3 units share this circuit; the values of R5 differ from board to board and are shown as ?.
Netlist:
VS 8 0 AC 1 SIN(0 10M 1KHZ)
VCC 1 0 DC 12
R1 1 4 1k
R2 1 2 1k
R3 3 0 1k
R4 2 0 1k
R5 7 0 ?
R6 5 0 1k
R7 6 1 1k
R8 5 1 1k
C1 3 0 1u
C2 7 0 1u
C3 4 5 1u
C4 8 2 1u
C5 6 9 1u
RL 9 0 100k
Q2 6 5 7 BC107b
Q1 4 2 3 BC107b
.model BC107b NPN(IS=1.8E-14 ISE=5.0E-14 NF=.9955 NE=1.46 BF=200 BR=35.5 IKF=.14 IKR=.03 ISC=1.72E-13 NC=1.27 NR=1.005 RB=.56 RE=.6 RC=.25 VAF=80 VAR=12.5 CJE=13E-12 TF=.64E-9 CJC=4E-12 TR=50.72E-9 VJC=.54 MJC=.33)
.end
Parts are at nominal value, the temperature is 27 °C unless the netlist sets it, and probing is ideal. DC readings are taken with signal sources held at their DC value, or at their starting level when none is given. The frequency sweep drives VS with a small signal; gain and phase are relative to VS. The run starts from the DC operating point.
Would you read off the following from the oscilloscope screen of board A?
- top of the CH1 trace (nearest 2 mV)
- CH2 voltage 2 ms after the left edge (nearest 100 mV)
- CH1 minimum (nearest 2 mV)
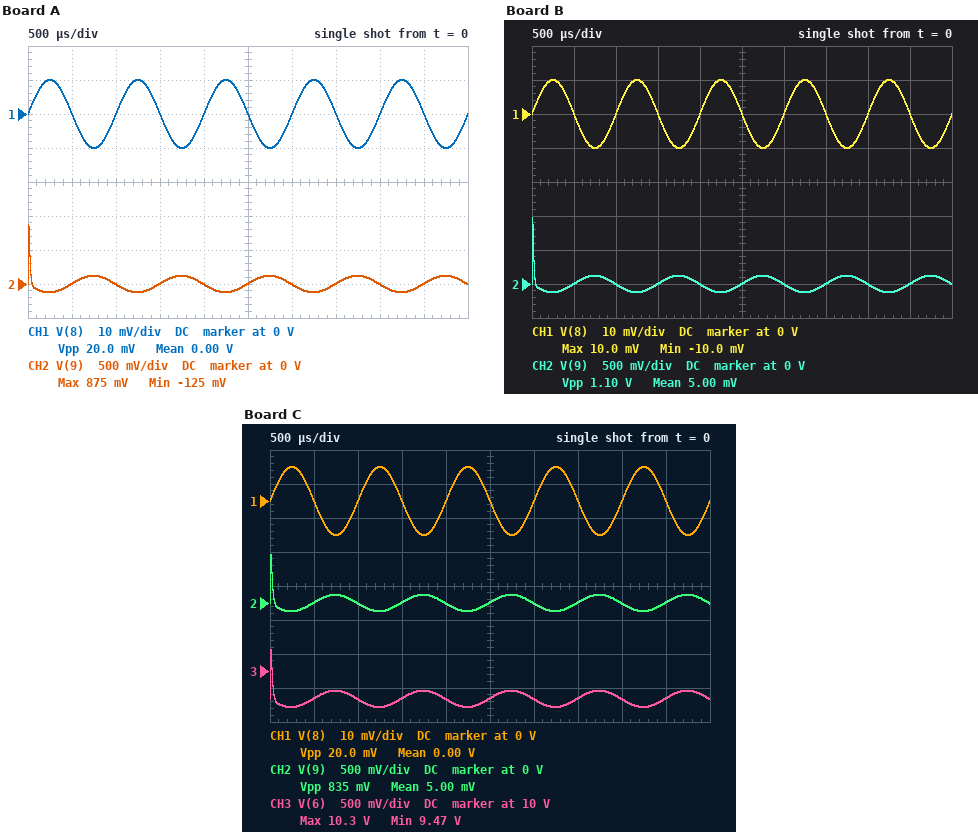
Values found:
10 mV
0 V
-10 mV
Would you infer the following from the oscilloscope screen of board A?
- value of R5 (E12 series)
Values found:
1.5 kΩ
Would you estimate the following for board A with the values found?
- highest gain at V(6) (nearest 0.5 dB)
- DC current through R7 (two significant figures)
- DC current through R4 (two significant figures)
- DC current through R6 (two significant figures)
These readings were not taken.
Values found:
74.5 dB
3.5 mA
6.0 mA
6.0 mA
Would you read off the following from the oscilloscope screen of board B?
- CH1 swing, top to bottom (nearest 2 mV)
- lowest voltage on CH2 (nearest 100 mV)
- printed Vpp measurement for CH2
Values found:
20 mV
-100 mV
1.10 V
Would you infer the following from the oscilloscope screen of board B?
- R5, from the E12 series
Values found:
1.2 kΩ
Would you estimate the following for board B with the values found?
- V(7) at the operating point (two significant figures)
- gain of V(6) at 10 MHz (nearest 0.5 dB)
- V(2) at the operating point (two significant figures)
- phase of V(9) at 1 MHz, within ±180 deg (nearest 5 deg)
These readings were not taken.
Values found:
5.3 V
58.0 dB
6.0 V
-35 deg
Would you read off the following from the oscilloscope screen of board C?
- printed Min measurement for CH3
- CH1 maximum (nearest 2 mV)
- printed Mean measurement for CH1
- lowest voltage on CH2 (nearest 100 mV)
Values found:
9.47 V
10 mV
0.00 V
-100 mV
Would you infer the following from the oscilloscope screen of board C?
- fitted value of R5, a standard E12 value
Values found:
2.2 kΩ
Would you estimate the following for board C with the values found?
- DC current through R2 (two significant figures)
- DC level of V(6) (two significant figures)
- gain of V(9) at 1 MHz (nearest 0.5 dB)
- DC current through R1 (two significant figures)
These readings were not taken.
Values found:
6.0 mA
9.6 V
71.5 dB
5.3 mA
